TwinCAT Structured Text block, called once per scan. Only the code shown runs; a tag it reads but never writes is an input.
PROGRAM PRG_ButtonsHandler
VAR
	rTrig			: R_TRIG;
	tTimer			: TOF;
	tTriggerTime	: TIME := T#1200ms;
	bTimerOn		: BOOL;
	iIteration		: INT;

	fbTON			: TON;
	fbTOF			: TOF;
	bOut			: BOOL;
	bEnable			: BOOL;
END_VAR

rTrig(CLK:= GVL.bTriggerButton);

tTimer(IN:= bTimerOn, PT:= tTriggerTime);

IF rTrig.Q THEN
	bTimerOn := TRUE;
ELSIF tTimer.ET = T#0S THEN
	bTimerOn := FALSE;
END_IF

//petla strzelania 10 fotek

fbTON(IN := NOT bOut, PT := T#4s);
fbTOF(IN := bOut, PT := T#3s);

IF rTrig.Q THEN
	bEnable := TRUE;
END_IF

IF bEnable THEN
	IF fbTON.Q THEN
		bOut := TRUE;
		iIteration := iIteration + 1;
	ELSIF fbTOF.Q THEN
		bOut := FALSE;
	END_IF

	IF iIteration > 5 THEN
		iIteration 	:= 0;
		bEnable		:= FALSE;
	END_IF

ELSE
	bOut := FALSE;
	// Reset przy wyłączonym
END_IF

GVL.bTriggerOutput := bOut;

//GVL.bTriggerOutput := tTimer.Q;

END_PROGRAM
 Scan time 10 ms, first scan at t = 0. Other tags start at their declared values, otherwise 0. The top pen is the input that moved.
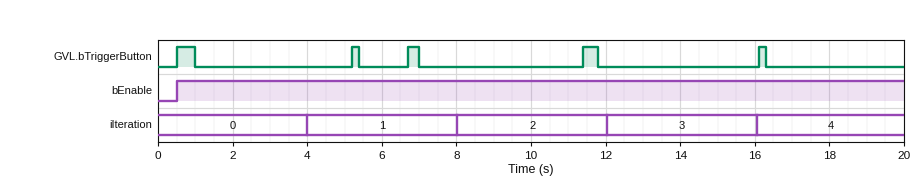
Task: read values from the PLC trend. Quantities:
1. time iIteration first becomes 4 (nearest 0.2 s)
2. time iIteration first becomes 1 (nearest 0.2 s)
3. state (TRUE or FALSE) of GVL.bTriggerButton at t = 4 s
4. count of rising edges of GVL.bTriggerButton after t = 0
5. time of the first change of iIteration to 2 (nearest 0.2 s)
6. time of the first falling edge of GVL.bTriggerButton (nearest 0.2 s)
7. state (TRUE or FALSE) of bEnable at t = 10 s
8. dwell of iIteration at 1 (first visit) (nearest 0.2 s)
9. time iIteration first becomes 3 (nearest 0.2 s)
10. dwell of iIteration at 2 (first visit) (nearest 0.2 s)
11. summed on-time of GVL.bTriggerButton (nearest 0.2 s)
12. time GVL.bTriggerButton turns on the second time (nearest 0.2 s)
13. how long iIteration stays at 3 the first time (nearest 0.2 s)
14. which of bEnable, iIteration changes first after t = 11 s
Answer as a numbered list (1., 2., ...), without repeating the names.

1. 16.0 s
2. 4.0 s
3. FALSE
4. 5
5. 8.0 s
6. 1.0 s
7. TRUE
8. 4.0 s
9. 12.0 s
10. 4.0 s
11. 1.6 s
12. 5.2 s
13. 4.0 s
14. iIteration
